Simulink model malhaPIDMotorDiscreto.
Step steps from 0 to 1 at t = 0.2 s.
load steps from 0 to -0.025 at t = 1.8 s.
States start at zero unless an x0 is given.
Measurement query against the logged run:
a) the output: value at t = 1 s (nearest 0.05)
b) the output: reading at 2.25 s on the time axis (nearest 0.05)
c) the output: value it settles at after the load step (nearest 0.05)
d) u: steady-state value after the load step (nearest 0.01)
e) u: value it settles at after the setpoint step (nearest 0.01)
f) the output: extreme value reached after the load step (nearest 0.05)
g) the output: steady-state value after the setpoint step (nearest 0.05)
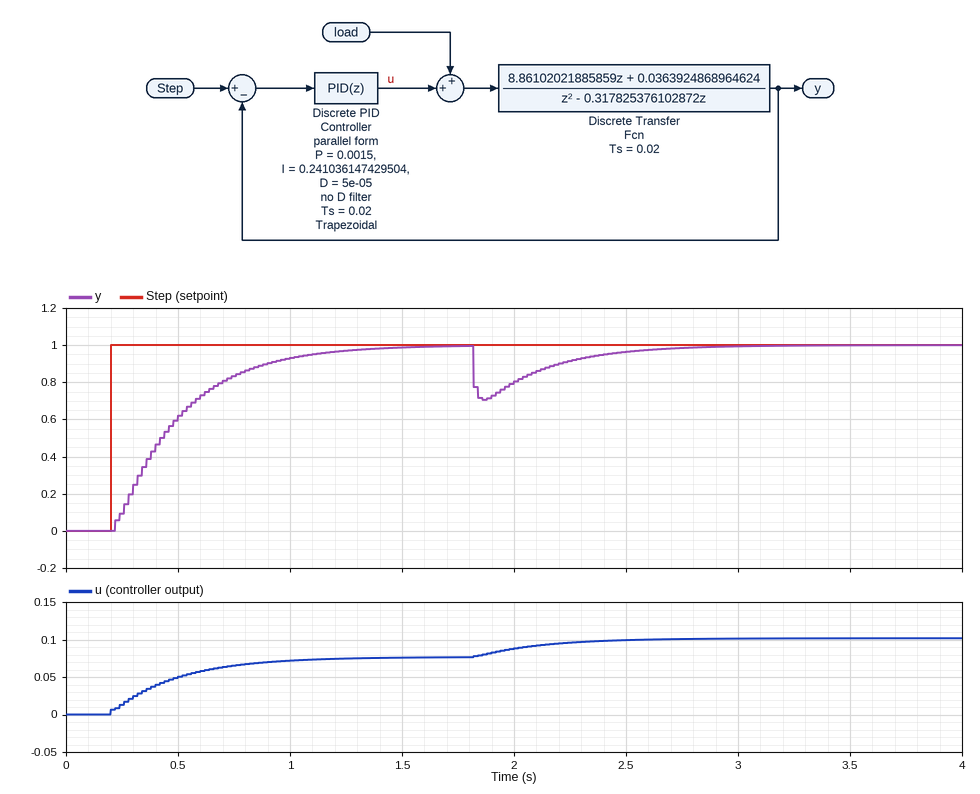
0.95
0.90
1.00
0.10
0.08
0.70
1.00
